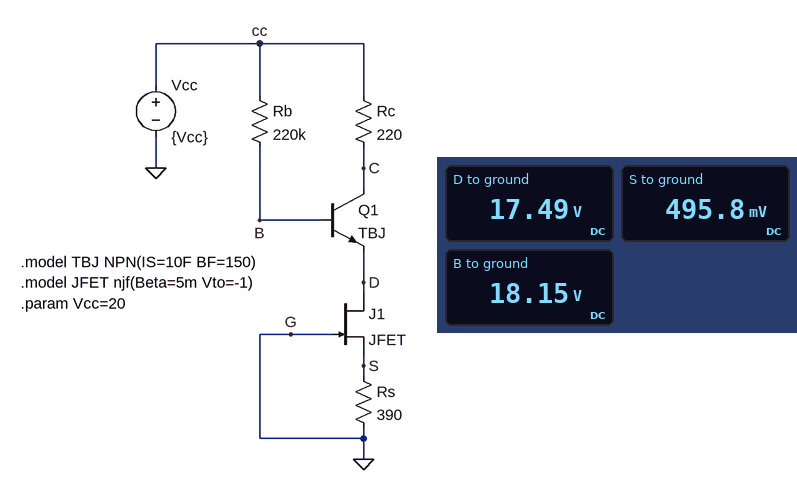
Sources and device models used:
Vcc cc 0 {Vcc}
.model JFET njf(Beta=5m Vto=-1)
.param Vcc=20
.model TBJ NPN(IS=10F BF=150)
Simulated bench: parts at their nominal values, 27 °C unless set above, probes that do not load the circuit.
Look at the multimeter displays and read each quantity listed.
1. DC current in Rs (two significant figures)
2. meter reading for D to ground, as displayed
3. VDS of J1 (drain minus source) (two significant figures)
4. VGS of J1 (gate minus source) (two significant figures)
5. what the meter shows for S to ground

1.3 mA
17.49 V
17 V
-500 mV
495.8 mV
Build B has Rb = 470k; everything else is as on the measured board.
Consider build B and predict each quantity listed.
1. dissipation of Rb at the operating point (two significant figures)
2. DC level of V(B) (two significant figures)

33 µW
16 V
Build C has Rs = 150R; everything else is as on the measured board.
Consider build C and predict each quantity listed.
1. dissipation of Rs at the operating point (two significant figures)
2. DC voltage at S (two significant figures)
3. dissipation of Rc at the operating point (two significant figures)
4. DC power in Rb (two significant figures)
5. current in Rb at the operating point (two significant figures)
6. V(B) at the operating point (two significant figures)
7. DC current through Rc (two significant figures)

740 µW
330 mV
1.1 mW
48 µW
15 µA
17 V
2.2 mA
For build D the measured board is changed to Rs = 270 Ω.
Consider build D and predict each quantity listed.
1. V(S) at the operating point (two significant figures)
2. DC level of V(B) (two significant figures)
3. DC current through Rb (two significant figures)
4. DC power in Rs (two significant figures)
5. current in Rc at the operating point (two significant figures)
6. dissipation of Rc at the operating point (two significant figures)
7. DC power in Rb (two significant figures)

430 mV
18 V
11 µA
700 µW
1.6 mA
560 µW
25 µW
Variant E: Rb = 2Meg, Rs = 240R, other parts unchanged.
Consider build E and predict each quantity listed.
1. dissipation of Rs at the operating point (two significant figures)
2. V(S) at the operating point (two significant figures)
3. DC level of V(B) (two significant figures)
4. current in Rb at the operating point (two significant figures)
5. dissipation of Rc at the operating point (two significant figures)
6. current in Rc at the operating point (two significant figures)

480 µW
340 mV
1.3 V
9.4 µA
430 µW
1.4 mA
